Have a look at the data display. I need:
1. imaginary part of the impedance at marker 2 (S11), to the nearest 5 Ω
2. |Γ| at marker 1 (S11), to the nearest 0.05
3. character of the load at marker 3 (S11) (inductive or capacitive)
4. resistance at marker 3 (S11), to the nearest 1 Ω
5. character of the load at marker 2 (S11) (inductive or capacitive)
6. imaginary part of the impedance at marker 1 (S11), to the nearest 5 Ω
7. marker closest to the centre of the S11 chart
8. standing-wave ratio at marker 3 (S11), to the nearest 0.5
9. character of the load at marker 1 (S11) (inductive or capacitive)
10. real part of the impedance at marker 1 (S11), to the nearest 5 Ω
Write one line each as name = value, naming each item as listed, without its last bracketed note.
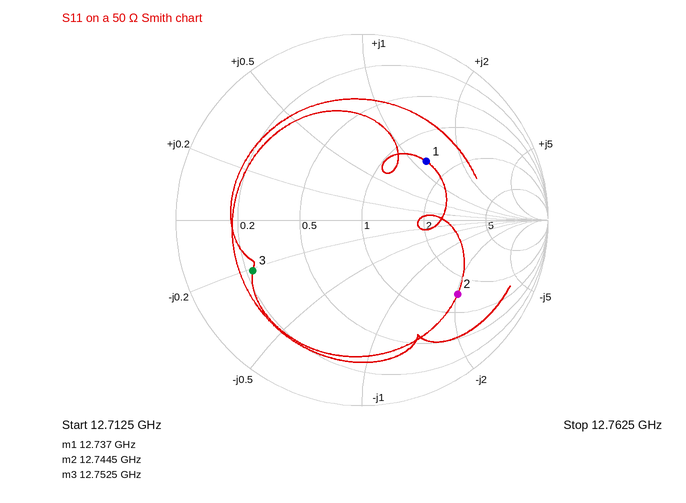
imaginary part of the impedance at marker 2 (S11), to the nearest 5 Ω = -100 Ω
|Γ| at marker 1 (S11), to the nearest 0.05 = 0.45
character of the load at marker 3 (S11) = capacitive
resistance at marker 3 (S11), to the nearest 1 Ω = 11 Ω
character of the load at marker 2 (S11) = capacitive
imaginary part of the impedance at marker 1 (S11), to the nearest 5 Ω = +60 Ω
marker closest to the centre of the S11 chart = marker 1
standing-wave ratio at marker 3 (S11), to the nearest 0.5 = 4.5
character of the load at marker 1 (S11) = inductive
real part of the impedance at marker 1 (S11), to the nearest 5 Ω = 75 Ω
